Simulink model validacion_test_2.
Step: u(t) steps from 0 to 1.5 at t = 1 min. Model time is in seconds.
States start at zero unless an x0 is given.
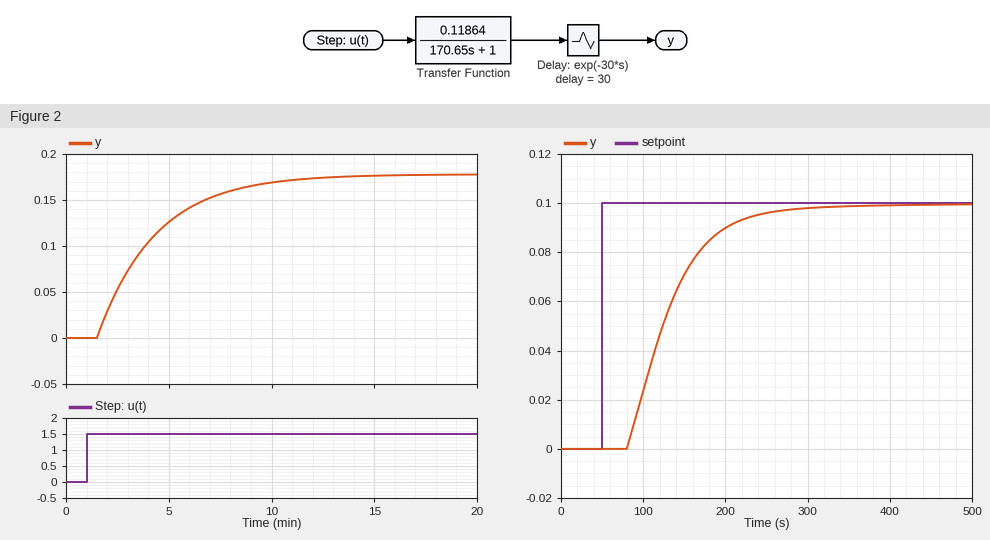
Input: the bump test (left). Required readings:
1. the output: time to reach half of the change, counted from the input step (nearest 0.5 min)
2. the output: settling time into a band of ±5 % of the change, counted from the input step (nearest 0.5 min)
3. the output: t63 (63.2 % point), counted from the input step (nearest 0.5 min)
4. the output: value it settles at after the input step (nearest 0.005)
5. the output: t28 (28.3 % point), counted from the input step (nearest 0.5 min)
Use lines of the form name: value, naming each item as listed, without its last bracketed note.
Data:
the output: time to reach half of the change, counted from the input step: 2.5 min
the output: settling time into a band of ±5 % of the change, counted from the input step: 9.0 min
the output: t63 (63.2 % point), counted from the input step: 3.5 min
the output: value it settles at after the input step: 0.180
the output: t28 (28.3 % point), counted from the input step: 1.5 min
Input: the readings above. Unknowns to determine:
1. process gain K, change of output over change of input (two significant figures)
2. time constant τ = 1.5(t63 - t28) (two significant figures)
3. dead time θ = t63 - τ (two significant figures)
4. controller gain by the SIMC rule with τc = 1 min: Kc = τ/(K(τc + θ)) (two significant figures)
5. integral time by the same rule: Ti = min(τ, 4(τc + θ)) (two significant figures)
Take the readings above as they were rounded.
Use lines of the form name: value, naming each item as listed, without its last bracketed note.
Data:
process gain K, change of output over change of input: 0.12
time constant τ = 1.5(t63 - t28): 3.0 min
dead time θ = t63 - τ: 0.50 min
controller gain by the SIMC rule with τc = 1 min: Kc = τ/(K(τc + θ)): 17
integral time by the same rule: Ti = min(τ, 4(τc + θ)): 3.0 min
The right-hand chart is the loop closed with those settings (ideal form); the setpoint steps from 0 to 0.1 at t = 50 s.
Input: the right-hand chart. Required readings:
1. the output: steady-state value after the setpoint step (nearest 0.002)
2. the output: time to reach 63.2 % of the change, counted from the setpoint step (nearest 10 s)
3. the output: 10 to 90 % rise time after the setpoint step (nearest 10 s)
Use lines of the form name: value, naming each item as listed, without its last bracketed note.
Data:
the output: steady-state value after the setpoint step: 0.100
the output: time to reach 63.2 % of the change, counted from the setpoint step: 90 s
the output: 10 to 90 % rise time after the setpoint step: 110 s
